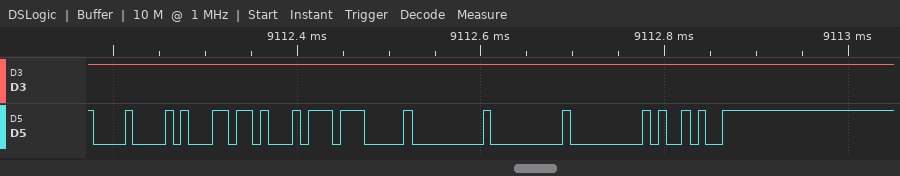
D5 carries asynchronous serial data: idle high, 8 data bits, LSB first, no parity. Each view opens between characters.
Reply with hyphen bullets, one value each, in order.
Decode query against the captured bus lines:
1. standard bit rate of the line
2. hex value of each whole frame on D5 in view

- 115200 baud
- 08, B1, D1, 07, 00, 00, 00, 29
